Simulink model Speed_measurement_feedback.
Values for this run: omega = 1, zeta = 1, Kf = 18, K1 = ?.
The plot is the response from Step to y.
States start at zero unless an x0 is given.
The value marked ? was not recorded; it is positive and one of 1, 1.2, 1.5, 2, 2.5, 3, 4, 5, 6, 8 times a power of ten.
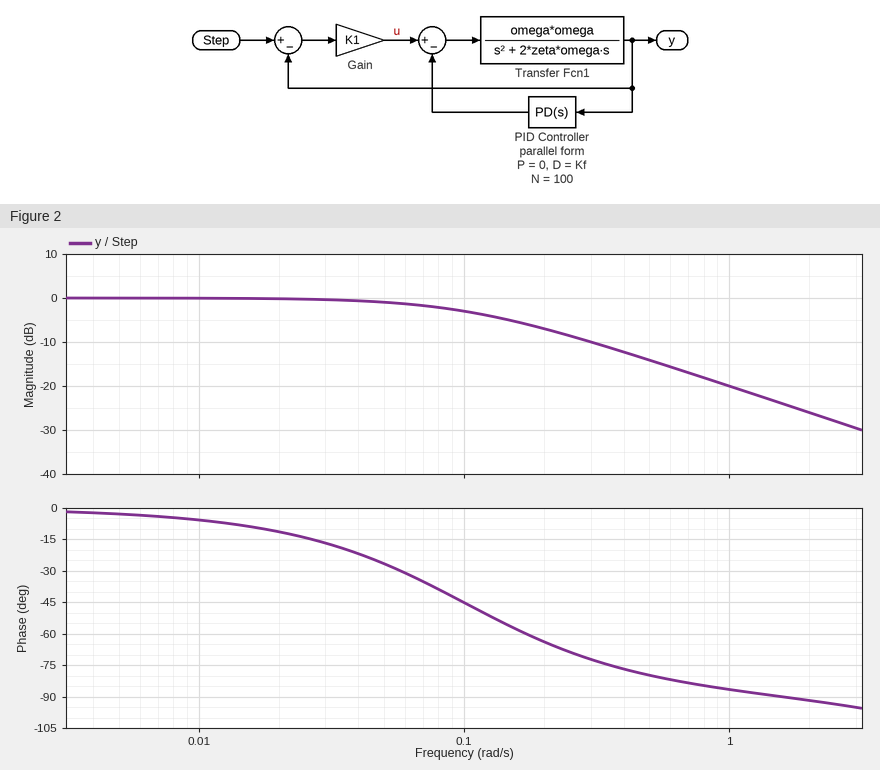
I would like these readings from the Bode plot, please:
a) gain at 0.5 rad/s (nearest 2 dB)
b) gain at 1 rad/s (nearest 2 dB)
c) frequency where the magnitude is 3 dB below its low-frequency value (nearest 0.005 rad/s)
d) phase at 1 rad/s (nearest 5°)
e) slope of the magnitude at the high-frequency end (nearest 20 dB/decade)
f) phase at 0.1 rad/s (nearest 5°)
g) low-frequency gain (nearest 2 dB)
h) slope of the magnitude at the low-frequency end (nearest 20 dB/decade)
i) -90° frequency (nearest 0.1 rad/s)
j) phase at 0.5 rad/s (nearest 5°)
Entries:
-14 dB
-20 dB
0.100 rad/s
-85°
-20 dB/decade
-45°
0 dB
0 dB/decade
1.6 rad/s
-80°
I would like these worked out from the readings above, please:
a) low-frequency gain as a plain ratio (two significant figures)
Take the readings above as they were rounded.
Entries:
1.0
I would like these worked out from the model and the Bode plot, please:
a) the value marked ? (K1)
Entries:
2
